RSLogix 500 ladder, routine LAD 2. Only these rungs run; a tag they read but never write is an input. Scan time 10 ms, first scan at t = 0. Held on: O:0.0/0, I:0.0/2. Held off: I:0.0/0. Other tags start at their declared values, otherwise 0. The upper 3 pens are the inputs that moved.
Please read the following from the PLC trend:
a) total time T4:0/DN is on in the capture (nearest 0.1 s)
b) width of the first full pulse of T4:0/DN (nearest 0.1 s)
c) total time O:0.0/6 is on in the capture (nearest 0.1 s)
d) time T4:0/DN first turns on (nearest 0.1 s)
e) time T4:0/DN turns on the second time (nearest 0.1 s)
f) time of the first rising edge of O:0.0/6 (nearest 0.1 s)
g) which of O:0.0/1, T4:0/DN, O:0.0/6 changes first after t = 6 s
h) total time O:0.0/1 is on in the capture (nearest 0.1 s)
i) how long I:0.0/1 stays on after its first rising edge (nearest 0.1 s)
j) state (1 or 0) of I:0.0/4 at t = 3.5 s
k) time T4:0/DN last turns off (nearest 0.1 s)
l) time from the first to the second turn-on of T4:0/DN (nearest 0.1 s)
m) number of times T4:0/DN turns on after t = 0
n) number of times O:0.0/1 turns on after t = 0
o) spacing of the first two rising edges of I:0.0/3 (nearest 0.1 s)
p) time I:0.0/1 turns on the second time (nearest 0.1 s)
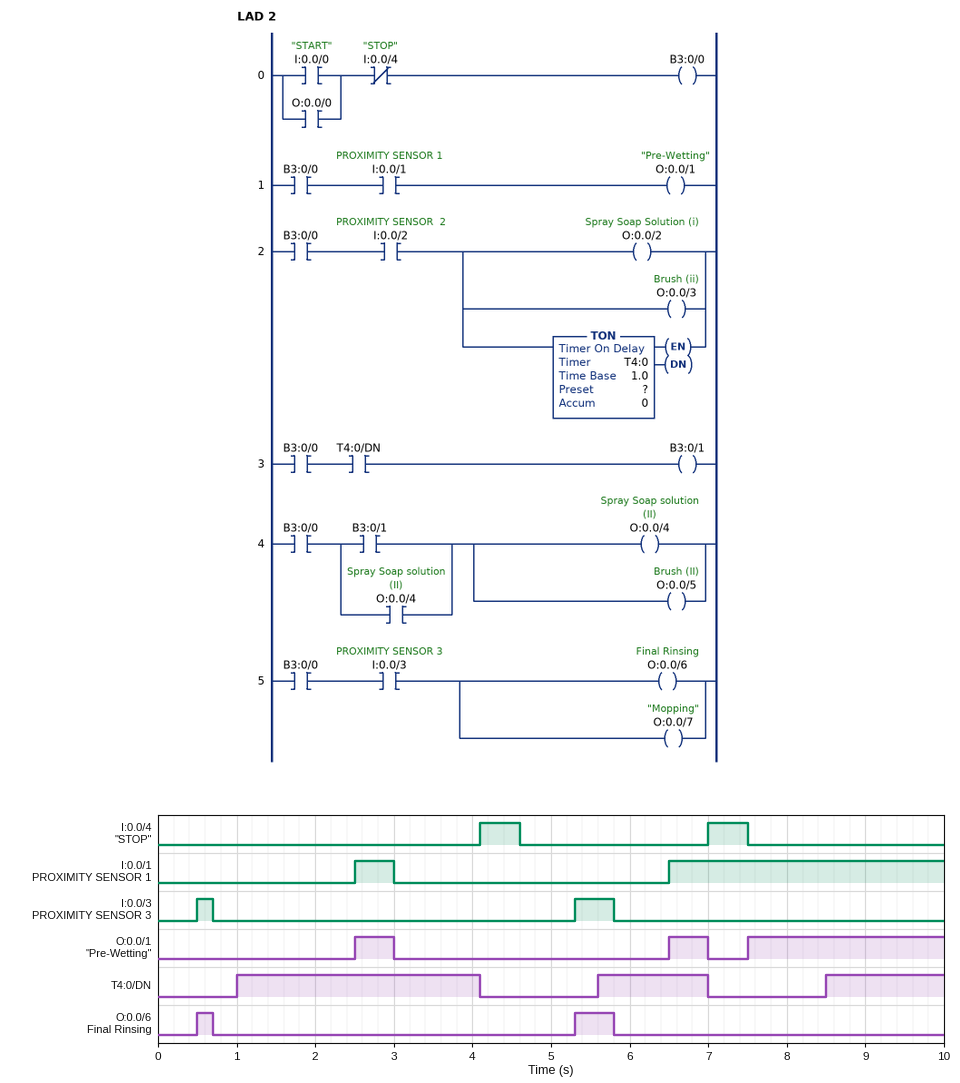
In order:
6.0 s
3.1 s
0.7 s
1.0 s
5.6 s
0.5 s
O:0.0/1
3.5 s
0.5 s
0
7.0 s
4.6 s
3
3
4.8 s
6.5 s
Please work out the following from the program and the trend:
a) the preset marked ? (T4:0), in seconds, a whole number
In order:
1 s
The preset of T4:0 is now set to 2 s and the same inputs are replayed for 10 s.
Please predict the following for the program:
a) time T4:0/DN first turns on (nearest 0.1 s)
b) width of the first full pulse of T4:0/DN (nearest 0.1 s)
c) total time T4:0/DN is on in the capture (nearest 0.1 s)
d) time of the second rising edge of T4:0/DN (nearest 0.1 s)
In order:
2.0 s
2.1 s
3.0 s
6.6 s
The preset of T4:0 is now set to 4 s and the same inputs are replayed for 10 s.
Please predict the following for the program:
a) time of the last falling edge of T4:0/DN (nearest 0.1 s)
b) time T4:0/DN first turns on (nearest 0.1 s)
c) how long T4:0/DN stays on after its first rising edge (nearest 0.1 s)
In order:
4.1 s
4.0 s
0.1 s
